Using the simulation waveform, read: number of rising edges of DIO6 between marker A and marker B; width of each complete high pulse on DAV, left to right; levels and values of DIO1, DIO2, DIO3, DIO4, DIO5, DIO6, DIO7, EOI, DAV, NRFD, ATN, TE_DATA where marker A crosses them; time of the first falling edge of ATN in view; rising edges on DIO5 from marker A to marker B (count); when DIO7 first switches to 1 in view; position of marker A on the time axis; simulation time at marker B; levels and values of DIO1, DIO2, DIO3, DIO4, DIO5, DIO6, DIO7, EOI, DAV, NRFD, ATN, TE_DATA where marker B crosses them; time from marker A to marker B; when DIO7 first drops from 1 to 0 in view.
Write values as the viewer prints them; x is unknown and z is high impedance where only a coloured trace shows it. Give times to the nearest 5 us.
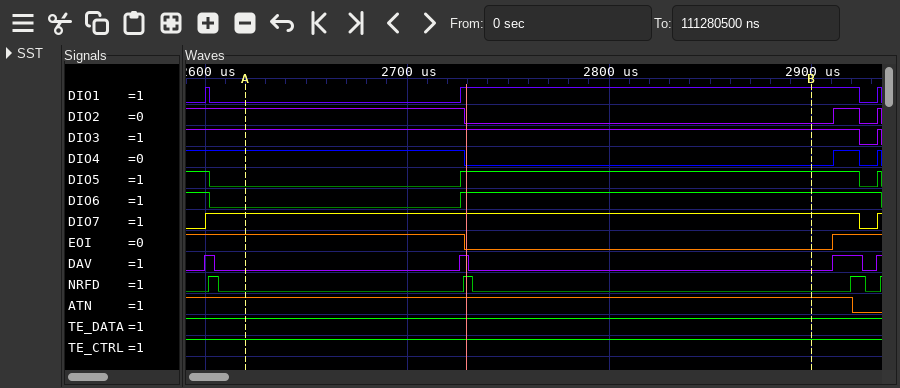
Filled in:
1
5 us, 5 us, 15 us
DIO1=0, DIO2=1, DIO3=1, DIO4=1, DIO5=0, DIO6=0, DIO7=1, EOI=1, DAV=0, NRFD=0, ATN=1, TE_DATA=1
2920 us
1
2600 us
2620 us
2900 us
DIO1=1, DIO2=0, DIO3=1, DIO4=0, DIO5=1, DIO6=1, DIO7=1, EOI=0, DAV=0, NRFD=0, ATN=1, TE_DATA=1
280 us
2925 us
